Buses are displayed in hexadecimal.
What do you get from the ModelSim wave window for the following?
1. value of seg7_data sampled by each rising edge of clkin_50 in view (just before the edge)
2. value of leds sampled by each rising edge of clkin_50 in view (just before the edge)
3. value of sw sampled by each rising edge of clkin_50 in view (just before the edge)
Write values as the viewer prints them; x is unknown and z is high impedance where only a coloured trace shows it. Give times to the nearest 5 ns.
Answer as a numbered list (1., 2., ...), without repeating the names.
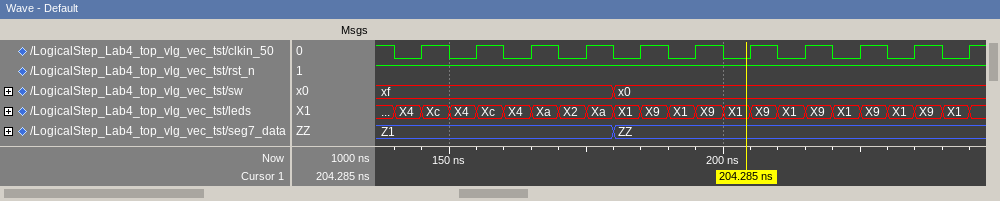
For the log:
1. Z1, Z1, Z1, Z1, ZZ, ZZ, ZZ, ZZ, ZZ, ZZ, ZZ
2. X4, X4, X4, X2, X1, X1, X1, X1, X1, X1, X1
3. xf, xf, xf, xf, x0, x0, x0, x0, x0, x0, x0
